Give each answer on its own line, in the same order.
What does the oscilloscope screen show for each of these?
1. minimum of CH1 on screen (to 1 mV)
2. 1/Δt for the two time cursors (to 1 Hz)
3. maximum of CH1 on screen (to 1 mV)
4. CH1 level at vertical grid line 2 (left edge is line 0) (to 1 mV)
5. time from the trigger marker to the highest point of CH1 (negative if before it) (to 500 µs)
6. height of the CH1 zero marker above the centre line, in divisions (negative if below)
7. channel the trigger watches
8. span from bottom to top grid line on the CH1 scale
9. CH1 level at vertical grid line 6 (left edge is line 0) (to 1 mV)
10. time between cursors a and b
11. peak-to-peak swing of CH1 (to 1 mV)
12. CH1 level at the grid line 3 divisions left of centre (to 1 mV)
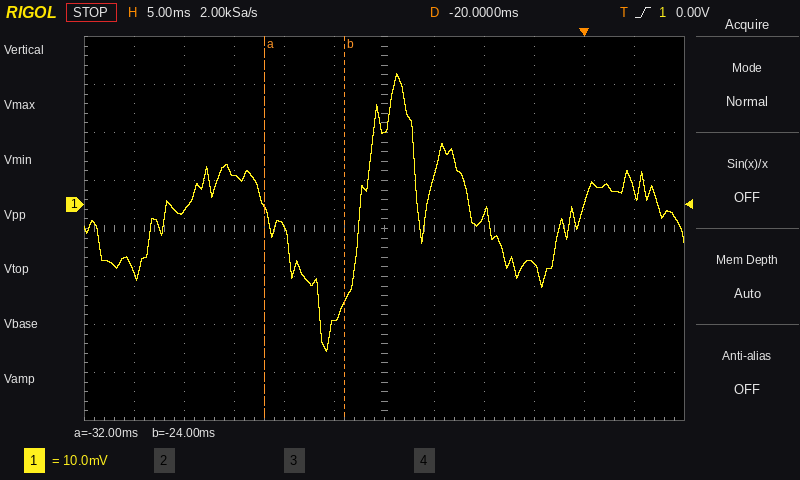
-31 mV
125 Hz
27 mV
-1 mV
-18.5 ms
+0.5 div
CH1
80 mV
15 mV
8.0 ms
58 mV
6 mV
